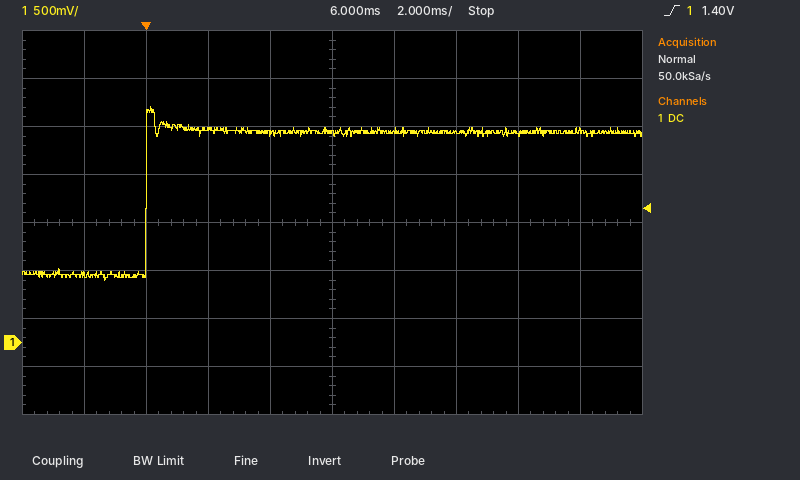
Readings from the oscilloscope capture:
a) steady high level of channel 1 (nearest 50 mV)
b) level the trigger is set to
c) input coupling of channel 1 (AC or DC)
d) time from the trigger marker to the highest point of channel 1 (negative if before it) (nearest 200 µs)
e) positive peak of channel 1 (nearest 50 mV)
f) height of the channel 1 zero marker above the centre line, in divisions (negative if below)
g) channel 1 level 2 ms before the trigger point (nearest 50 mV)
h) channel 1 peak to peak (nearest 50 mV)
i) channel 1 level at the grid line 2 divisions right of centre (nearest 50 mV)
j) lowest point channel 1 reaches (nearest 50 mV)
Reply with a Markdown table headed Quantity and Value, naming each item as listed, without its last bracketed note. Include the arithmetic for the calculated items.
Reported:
| Quantity | Value |
|---|---|
| steady high level of channel 1 | 2.20 V |
| level the trigger is set to | 1.40 V |
| input coupling of channel 1 | DC |
| time from the trigger marker to the highest point of channel 1 (negative if before it) | +200 µs |
| positive peak of channel 1 | 2.45 V |
| height of the channel 1 zero marker above the centre line, in divisions | -2.5 div |
| channel 1 level 2 ms before the trigger point | 700 mV |
| channel 1 peak to peak | 2.45 V − (650 mV) = 1.80 V |
| channel 1 level at the grid line 2 divisions right of centre | 2.20 V |
| lowest point channel 1 reaches | 650 mV |
